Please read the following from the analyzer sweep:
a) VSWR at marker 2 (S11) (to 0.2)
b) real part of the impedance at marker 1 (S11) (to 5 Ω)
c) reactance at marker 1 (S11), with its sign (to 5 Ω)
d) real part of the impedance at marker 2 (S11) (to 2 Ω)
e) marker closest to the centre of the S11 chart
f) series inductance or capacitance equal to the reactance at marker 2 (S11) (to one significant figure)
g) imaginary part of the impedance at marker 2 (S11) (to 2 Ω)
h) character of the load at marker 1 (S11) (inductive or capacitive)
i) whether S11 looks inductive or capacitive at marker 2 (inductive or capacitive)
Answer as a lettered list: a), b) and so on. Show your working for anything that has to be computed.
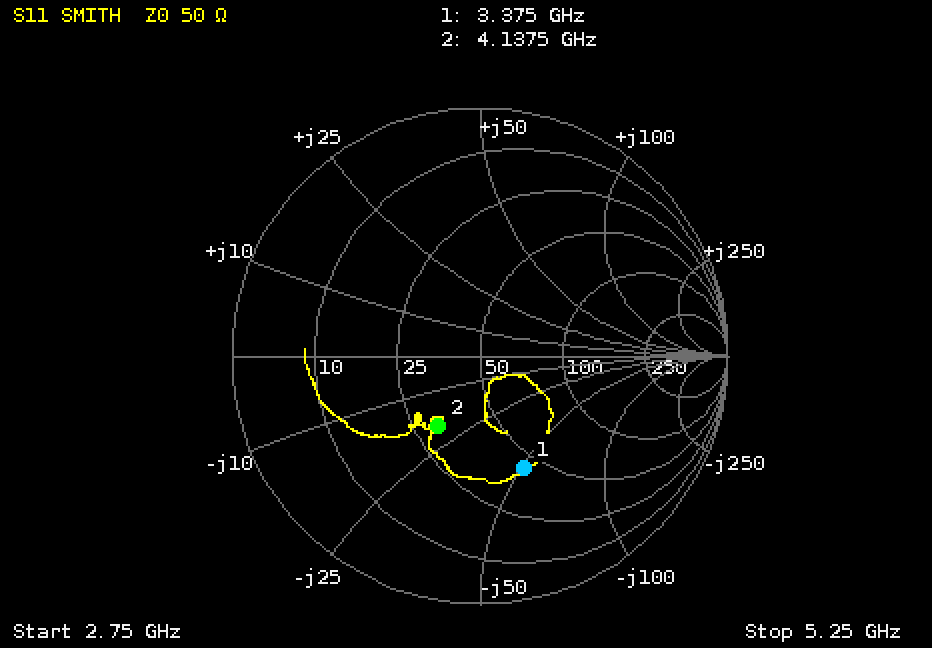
a) 2.0
b) 45 Ω
c) -50 Ω
d) 30 Ω
e) marker 2
f) C = 1/(2π × 4.1375 GHz × 20 Ω) ≈ 2 pF
g) -20 Ω
h) capacitive
i) capacitive
